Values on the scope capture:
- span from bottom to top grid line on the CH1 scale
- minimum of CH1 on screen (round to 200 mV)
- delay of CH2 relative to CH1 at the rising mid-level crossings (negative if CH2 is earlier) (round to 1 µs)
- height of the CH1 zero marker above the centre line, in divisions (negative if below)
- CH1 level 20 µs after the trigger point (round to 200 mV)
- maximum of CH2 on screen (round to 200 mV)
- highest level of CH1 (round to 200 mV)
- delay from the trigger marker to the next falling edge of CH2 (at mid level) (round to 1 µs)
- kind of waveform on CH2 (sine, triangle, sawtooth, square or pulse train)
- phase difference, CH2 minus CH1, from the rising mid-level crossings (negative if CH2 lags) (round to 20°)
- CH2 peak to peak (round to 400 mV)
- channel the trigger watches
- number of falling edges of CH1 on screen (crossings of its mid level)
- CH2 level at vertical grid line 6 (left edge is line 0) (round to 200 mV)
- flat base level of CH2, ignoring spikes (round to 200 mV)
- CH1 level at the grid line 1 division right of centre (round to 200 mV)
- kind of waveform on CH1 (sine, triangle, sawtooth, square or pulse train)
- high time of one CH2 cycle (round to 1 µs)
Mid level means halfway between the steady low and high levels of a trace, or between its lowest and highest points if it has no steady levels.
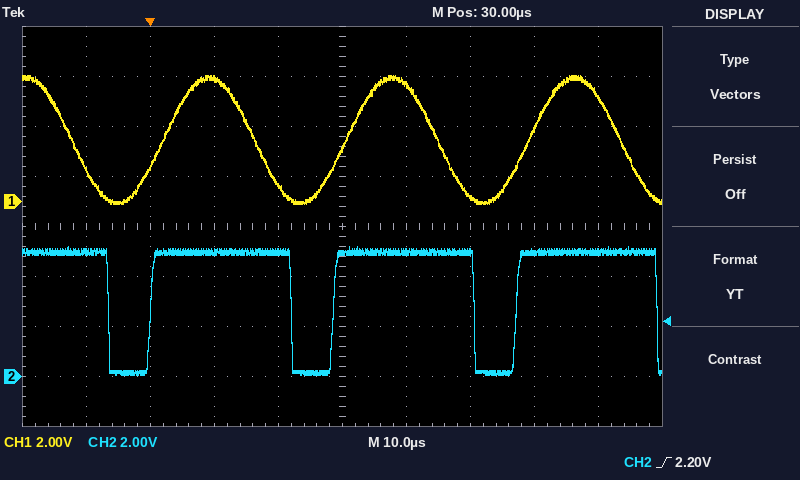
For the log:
16 V
0.0 V
-2 µs
+0.5 div
600 mV
5.2 V
5.0 V
22 µs
pulse train
+20°
5.2 V
CH2
4
5.0 V
200 mV
4.6 V
sine
22 µs
